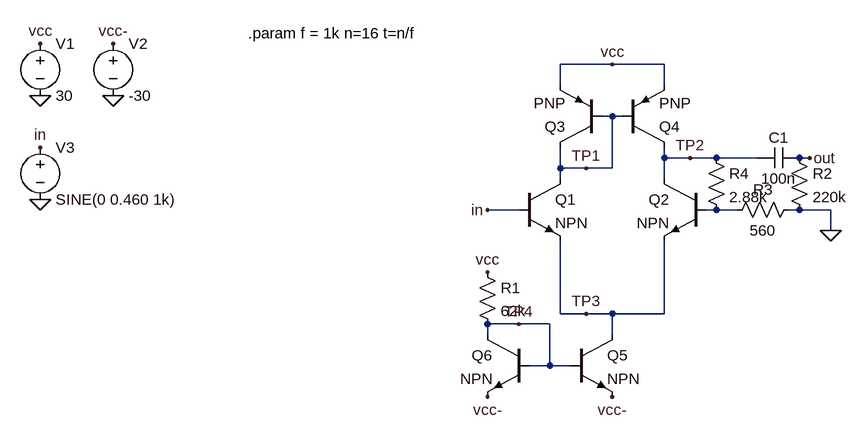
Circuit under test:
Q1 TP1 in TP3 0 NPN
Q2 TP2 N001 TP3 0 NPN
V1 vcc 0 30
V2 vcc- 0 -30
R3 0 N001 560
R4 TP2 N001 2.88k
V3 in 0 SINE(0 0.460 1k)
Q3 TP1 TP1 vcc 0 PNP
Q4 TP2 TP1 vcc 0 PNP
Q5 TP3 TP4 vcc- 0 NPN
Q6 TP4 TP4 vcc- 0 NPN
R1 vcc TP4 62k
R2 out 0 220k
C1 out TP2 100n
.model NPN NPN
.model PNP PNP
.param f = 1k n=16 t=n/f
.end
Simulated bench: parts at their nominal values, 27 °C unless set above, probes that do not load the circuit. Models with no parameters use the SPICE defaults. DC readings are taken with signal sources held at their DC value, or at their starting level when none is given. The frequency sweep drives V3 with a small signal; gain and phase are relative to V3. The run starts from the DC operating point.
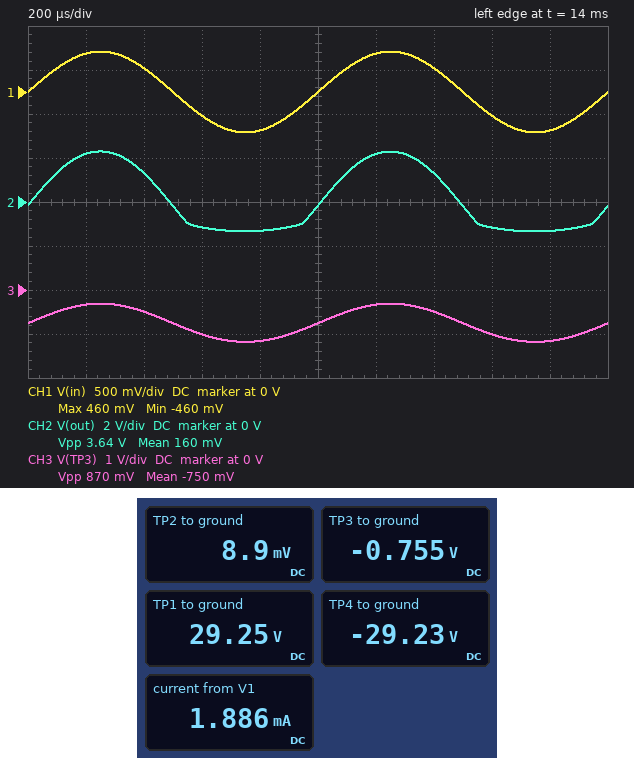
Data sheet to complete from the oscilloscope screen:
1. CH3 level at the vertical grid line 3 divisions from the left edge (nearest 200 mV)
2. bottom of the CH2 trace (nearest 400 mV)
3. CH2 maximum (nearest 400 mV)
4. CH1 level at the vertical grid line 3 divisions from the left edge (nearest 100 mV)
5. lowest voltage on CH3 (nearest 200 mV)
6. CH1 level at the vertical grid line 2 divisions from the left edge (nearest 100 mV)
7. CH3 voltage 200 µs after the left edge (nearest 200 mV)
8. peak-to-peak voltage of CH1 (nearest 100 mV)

-1.0 V
-1.2 V
2.4 V
-300 mV
-1.2 V
300 mV
-400 mV
900 mV
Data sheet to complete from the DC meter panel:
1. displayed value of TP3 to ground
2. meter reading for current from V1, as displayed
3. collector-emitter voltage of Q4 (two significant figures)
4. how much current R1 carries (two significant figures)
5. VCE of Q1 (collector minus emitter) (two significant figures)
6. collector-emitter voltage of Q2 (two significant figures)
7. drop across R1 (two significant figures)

-0.755 V
1.886 mA
-30 V
960 µA
30 V
760 mV
59 V
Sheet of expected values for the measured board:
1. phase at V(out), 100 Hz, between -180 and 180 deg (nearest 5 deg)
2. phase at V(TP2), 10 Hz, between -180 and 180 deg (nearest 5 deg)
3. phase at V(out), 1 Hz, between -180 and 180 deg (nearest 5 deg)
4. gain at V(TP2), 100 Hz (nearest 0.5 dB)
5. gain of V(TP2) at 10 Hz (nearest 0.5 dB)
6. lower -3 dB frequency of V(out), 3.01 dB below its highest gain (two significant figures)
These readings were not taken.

5 deg
0 deg
80 deg
15.0 dB
15.0 dB
7.2 Hz
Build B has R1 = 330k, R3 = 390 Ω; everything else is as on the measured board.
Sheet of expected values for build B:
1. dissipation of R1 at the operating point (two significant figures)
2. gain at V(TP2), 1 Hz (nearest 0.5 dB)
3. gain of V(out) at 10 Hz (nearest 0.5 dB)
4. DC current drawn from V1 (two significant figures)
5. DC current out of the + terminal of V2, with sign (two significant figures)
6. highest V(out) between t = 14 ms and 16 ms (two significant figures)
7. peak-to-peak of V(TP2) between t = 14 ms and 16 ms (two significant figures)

11 mW
13.5 dB
11.5 dB
350 µA
-360 µA
550 mV
1.1 V
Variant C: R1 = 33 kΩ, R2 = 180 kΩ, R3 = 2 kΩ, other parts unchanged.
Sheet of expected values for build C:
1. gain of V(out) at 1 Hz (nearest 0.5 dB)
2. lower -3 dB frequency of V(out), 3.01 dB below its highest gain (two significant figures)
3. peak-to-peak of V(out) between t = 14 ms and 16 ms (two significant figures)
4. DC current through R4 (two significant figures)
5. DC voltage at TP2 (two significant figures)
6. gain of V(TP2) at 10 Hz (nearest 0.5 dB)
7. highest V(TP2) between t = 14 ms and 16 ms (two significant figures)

-11.5 dB
8.8 Hz
2.2 V
8.2 µA
23 mV
7.5 dB
1.1 V
